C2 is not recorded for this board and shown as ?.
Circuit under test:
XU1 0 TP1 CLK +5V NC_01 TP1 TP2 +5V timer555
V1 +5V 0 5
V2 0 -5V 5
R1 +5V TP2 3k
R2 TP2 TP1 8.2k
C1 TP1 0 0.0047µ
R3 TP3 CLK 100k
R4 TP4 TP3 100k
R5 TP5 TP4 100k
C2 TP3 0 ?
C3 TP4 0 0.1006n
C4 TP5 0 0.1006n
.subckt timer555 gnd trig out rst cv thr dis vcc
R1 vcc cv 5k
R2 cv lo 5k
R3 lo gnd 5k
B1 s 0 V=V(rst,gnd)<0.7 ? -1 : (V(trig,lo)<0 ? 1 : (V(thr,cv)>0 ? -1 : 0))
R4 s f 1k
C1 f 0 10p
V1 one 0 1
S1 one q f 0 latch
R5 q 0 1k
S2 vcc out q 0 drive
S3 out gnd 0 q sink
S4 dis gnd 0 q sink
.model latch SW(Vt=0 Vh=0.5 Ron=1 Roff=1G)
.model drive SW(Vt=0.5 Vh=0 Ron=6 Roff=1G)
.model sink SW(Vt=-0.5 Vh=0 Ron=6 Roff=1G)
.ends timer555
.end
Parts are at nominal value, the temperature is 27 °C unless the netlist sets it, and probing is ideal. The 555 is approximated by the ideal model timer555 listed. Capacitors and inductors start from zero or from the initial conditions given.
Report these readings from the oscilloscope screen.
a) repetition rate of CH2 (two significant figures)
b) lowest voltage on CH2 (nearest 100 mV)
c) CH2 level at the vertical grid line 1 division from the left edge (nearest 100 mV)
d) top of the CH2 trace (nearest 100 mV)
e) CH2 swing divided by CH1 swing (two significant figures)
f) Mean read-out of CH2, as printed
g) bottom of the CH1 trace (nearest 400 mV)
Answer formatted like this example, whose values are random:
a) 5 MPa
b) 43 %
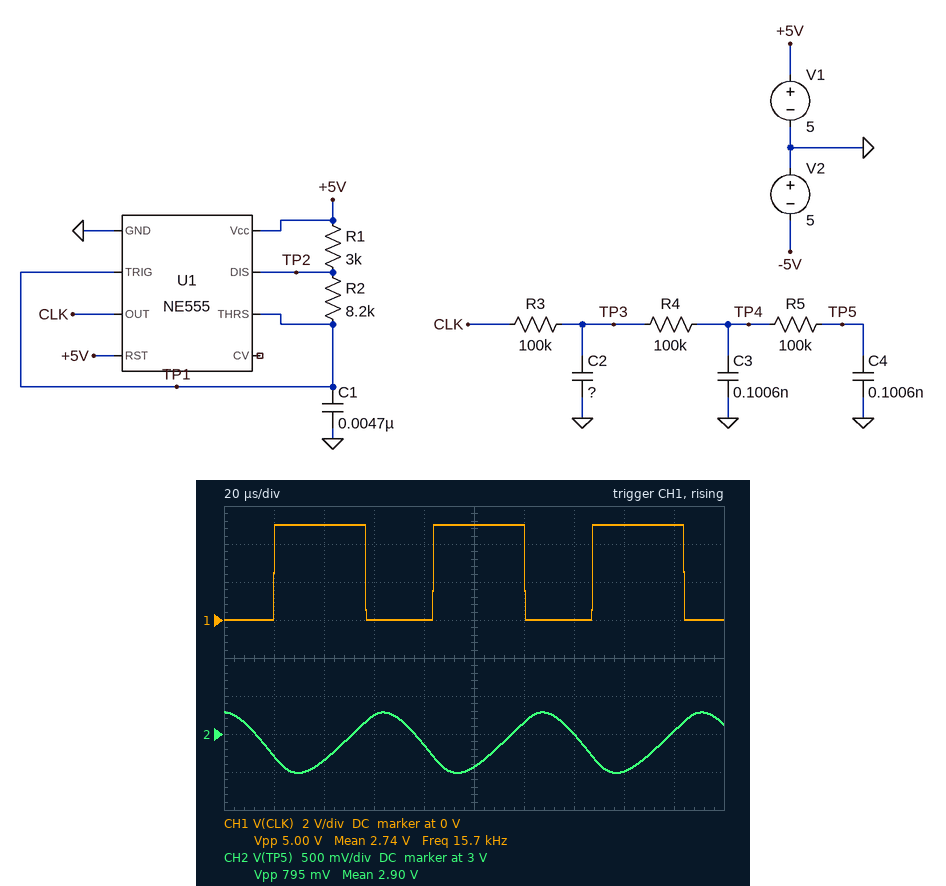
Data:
a) 16 kHz
b) 2.5 V
c) 2.7 V
d) 3.3 V
e) 0.16
f) 2.90 V
g) 0 V
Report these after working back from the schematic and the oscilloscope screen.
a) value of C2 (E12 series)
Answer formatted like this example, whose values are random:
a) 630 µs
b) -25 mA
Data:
a) 180 pF
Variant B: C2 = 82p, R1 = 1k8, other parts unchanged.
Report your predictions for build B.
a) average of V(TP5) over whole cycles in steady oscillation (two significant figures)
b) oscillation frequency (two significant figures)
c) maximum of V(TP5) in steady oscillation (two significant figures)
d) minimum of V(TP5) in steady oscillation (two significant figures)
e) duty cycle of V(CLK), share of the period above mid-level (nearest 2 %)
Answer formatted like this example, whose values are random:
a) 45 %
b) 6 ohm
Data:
a) 2.7 V
b) 17 kHz
c) 3.2 V
d) 2.2 V
e) 54 %
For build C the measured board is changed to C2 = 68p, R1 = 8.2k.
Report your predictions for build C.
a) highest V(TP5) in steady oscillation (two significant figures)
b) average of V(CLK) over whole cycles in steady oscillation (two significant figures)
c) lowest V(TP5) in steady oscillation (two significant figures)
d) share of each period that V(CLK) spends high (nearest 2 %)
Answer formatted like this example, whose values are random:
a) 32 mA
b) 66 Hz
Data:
a) 4.0 V
b) 3.3 V
c) 2.6 V
d) 66 %
